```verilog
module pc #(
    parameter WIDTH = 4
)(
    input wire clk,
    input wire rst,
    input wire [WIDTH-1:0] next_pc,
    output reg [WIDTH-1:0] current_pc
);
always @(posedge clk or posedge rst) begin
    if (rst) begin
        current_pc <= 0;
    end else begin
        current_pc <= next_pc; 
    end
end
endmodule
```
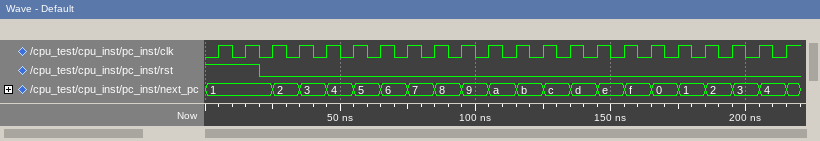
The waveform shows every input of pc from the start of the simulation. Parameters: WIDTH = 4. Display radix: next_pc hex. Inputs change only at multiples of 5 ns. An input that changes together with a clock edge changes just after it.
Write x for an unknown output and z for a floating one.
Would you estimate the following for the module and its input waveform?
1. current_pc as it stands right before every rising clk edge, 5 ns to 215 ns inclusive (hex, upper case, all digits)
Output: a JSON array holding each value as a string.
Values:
["0, 0, 0, 1, 2, 3, 4, 5, 6, 7, 8, 9, A, B, C, D, E, F, 0, 1, 2, 3"]
